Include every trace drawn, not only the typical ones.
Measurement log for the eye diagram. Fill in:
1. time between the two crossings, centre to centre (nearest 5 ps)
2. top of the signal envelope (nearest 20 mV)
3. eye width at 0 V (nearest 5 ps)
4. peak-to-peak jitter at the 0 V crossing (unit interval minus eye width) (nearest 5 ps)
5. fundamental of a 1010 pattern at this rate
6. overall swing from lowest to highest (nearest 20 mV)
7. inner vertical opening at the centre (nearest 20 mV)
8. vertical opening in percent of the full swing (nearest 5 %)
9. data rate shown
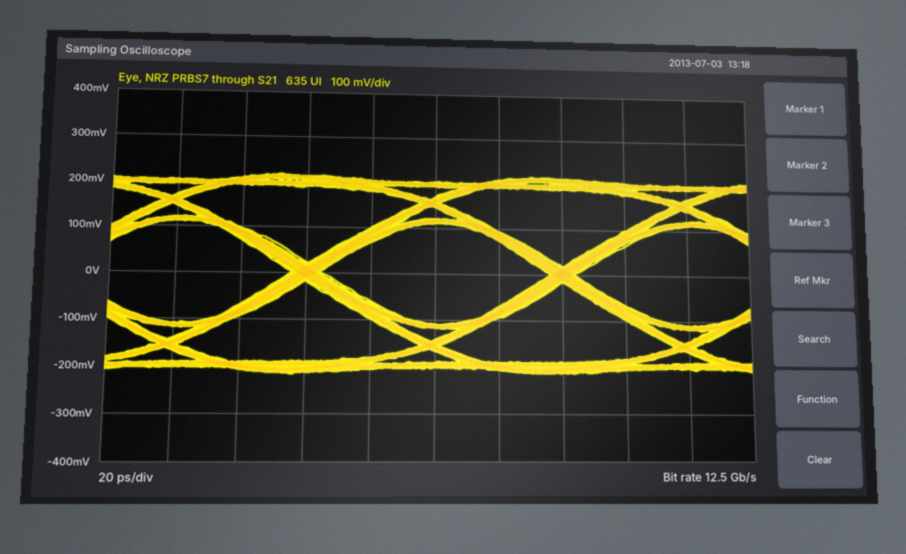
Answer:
80 ps
220 mV
70 ps
10 ps
6.25 GHz
440 mV
220 mV
50 %
12.5 Gb/s
